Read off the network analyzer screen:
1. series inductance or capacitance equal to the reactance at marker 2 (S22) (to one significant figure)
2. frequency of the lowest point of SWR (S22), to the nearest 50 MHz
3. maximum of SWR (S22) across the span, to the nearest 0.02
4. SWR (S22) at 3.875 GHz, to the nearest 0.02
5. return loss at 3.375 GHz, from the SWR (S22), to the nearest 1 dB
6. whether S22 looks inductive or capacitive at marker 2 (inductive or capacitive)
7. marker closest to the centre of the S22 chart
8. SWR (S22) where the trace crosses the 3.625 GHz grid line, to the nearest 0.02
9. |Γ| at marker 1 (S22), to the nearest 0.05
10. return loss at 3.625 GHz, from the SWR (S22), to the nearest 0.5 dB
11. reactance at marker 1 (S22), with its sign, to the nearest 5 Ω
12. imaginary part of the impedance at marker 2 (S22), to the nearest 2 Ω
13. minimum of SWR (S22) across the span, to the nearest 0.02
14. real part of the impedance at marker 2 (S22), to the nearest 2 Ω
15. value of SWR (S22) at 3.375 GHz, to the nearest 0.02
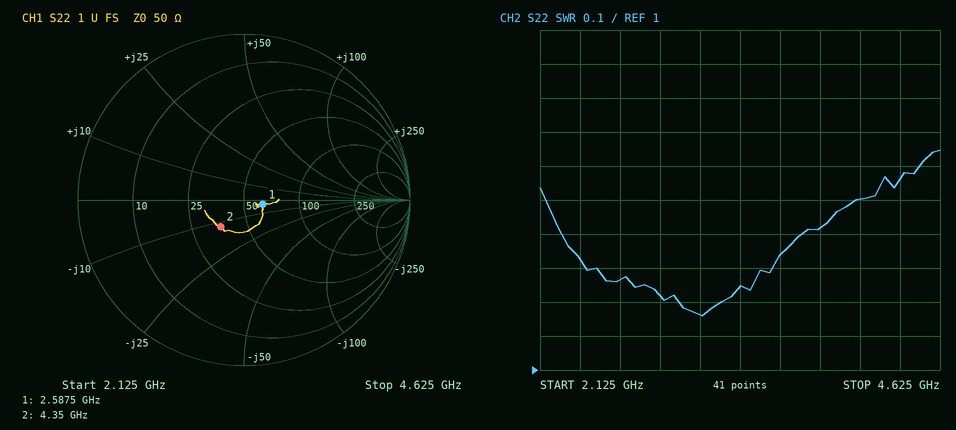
3 pF
3.15 GHz
1.64
1.42
19 dB
capacitive
marker 1
1.34
0.10
17.0 dB
-5 Ω
-12 Ω
1.16
36 Ω
1.24
